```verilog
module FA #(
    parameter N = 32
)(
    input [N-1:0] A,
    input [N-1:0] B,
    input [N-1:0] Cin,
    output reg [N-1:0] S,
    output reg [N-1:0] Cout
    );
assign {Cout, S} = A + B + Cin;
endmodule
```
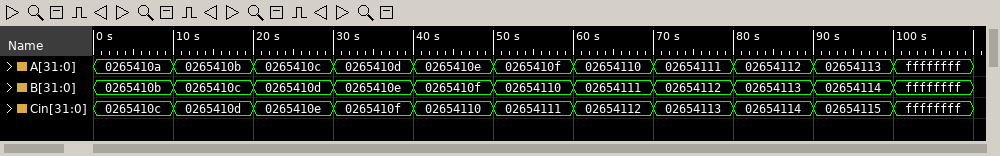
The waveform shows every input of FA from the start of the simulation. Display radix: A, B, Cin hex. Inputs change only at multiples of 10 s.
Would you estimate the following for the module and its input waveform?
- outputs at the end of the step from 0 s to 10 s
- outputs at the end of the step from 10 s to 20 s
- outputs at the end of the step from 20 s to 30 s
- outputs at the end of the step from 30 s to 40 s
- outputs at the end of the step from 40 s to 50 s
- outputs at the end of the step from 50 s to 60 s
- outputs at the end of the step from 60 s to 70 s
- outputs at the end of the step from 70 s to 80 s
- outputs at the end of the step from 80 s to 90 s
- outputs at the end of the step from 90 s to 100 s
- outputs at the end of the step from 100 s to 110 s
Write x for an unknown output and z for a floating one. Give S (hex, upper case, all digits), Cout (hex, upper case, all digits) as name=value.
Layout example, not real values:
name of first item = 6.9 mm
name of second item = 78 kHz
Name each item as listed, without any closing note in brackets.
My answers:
outputs at the end of the step from 0 s to 10 s = S=072FC321, Cout=00000000
outputs at the end of the step from 10 s to 20 s = S=072FC324, Cout=00000000
outputs at the end of the step from 20 s to 30 s = S=072FC327, Cout=00000000
outputs at the end of the step from 30 s to 40 s = S=072FC32A, Cout=00000000
outputs at the end of the step from 40 s to 50 s = S=072FC32D, Cout=00000000
outputs at the end of the step from 50 s to 60 s = S=072FC330, Cout=00000000
outputs at the end of the step from 60 s to 70 s = S=072FC333, Cout=00000000
outputs at the end of the step from 70 s to 80 s = S=072FC336, Cout=00000000
outputs at the end of the step from 80 s to 90 s = S=072FC339, Cout=00000000
outputs at the end of the step from 90 s to 100 s = S=072FC33C, Cout=00000000
outputs at the end of the step from 100 s to 110 s = S=FFFFFFFD, Cout=00000002
